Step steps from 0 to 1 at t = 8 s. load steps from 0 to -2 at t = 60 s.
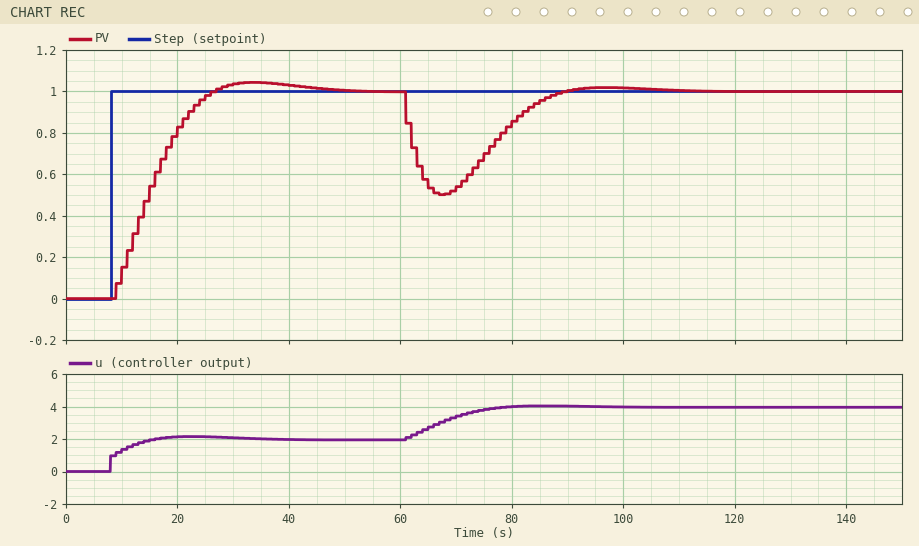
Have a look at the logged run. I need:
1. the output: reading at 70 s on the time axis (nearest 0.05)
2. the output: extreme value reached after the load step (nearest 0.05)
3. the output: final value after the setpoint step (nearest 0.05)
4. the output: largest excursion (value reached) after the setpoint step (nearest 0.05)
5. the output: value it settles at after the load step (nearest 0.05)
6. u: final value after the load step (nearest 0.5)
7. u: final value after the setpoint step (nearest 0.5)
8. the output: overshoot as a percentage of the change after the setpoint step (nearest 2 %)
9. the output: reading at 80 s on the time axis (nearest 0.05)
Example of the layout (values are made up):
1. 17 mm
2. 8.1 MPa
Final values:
1. 0.55
2. 0.50
3. 1.00
4. 1.05
5. 1.00
6. 4.0
7. 2.0
8. 4 %
9. 0.85
